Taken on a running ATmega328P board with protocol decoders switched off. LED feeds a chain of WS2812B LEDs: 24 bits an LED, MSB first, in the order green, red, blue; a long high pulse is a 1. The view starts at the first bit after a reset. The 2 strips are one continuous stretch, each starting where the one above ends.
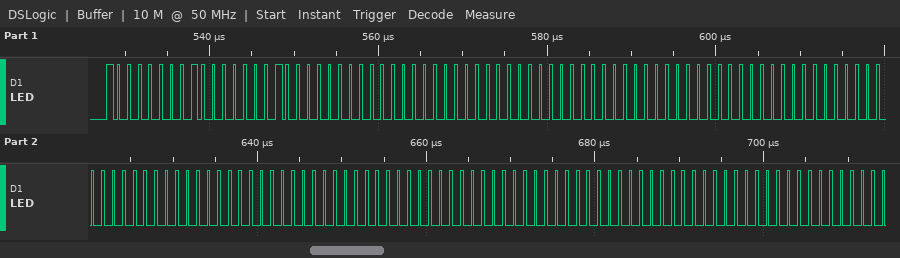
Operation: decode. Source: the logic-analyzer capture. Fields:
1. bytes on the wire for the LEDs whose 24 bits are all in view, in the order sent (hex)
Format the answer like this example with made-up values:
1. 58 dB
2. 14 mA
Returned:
1. 80 80 80 00 00 00 00 00 00 00 00 00 00 00 00 00 00 00
